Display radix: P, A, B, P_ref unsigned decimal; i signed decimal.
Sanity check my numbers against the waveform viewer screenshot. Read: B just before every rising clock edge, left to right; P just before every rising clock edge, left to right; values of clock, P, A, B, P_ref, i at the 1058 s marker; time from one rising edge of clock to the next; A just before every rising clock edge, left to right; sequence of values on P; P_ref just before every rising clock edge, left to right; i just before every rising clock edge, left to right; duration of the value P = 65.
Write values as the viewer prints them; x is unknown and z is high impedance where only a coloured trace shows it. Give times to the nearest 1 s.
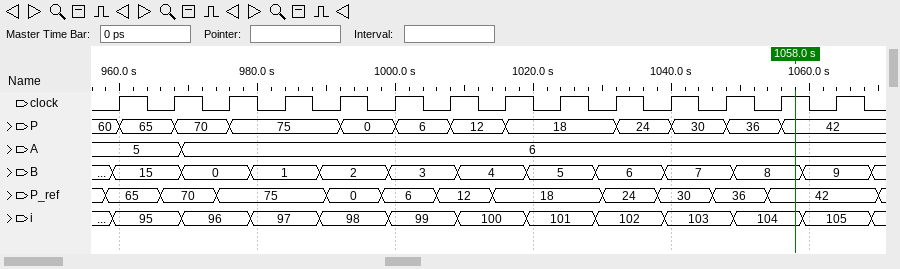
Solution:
15, 15, 0, 1, 2, 3, 3, 4, 5, 6, 7, 7, 8, 9
60, 65, 70, 75, 75, 0, 6, 12, 18, 18, 24, 30, 36, 42
clock=1, P=42, A=6, B=8, P_ref=42, i=104
8 s
5, 5, 6, 6, 6, 6, 6, 6, 6, 6, 6, 6, 6, 6
60, 65, 70, 75, 0, 6, 12, 18, 24, 30, 36, 42
65, 70, 75, 75, 0, 6, 12, 18, 18, 24, 30, 36, 42, 42
95, 95, 96, 97, 98, 99, 99, 100, 101, 102, 103, 103, 104, 105
8 s
